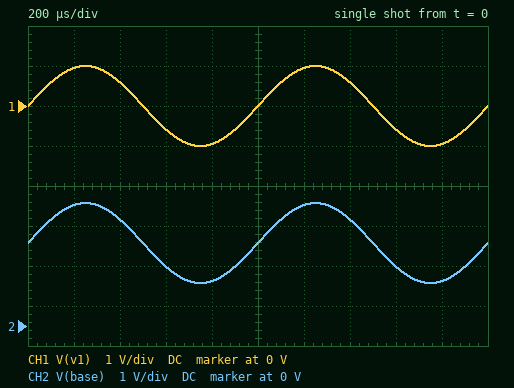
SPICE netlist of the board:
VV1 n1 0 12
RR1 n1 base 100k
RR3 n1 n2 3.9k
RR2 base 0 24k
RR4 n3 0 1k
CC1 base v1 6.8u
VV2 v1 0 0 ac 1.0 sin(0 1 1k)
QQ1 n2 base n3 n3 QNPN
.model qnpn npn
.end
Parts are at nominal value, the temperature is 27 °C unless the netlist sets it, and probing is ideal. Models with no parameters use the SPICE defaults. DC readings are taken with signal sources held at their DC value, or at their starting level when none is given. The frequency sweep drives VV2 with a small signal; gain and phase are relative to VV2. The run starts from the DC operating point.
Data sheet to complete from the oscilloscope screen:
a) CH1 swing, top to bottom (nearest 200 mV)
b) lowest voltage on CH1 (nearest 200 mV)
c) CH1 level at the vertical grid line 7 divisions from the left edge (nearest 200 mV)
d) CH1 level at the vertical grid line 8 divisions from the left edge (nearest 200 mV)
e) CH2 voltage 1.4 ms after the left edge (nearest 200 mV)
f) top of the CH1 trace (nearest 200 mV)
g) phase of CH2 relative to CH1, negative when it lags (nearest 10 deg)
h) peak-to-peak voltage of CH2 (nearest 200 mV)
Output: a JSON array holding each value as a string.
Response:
["2.0 V", "-1.0 V", "600 mV", "-600 mV", "2.6 V", "1.0 V", "0 deg", "2.0 V"]
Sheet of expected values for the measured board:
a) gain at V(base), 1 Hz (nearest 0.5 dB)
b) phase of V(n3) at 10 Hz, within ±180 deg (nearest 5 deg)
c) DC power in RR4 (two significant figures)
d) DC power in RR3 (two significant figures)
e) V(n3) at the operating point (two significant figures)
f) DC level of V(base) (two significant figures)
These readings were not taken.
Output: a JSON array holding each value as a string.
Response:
["-5.0 dB", "10 deg", "1.7 mW", "6.4 mW", "1.3 V", "2.1 V"]
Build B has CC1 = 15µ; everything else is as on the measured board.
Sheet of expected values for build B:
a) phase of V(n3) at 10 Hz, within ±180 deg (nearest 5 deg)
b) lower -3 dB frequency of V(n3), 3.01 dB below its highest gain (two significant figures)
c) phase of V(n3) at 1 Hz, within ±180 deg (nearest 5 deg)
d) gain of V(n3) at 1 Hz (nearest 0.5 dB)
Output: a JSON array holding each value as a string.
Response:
["5 deg", "650 mHz", "35 deg", "-1.5 dB"]
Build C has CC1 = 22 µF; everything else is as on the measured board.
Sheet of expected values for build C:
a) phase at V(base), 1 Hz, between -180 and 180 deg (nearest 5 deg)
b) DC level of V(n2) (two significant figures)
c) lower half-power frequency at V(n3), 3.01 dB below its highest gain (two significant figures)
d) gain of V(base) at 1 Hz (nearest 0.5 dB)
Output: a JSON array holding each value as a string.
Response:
["25 deg", "7.0 V", "440 mHz", "-1.0 dB"]
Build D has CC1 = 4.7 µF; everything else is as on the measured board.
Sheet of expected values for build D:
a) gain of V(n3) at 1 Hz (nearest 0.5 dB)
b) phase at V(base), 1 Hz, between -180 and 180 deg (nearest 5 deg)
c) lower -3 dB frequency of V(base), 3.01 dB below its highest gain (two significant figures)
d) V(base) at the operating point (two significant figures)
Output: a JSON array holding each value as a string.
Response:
["-7.5 dB", "65 deg", "2.1 Hz", "2.1 V"]
